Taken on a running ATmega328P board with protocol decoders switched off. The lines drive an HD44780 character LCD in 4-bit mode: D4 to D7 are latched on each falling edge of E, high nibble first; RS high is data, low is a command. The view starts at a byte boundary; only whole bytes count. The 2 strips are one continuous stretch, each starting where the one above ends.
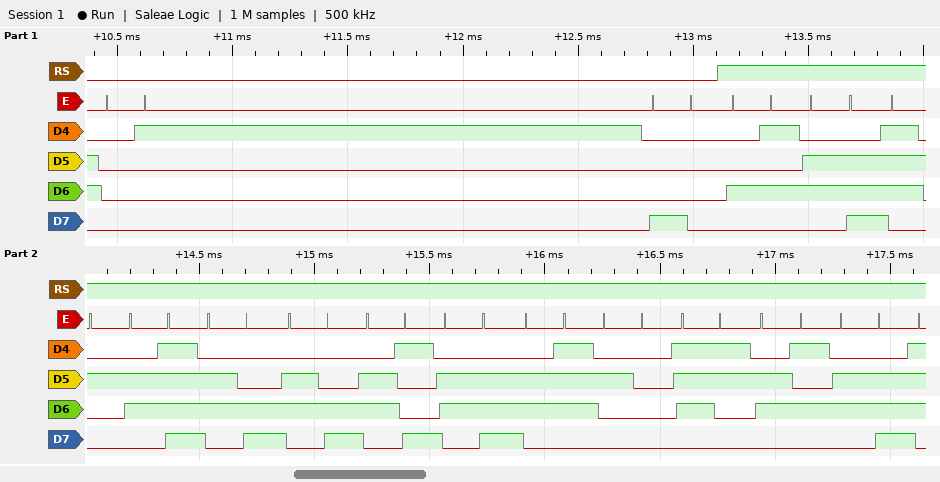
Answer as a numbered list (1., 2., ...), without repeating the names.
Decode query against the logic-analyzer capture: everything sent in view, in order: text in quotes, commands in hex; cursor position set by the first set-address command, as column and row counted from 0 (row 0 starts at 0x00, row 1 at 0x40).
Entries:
1. 0x01 0x80 "Enrolling sen"
2. column 0, row 0
